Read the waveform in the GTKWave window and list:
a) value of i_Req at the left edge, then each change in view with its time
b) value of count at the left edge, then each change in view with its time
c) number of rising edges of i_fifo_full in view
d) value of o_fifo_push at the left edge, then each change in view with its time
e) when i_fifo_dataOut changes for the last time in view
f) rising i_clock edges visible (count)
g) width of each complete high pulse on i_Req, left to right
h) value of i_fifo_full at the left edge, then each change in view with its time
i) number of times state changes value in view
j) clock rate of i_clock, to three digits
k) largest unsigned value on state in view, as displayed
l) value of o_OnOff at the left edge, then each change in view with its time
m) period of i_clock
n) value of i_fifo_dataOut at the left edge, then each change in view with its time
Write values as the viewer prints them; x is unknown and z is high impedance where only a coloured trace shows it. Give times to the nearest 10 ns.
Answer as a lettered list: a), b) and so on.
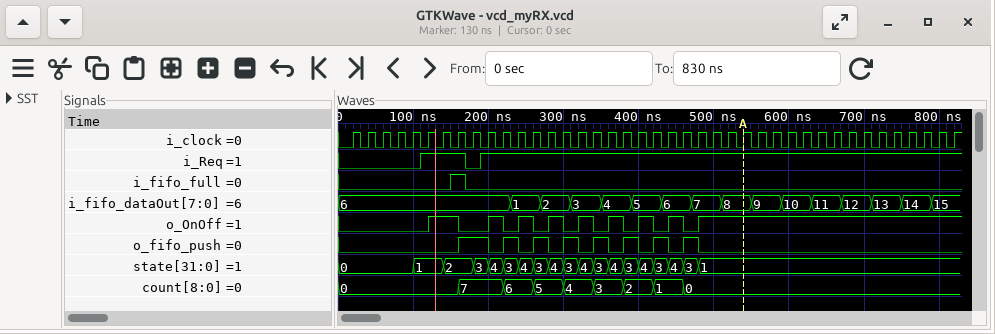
a) 0, 1 at 110 ns, 0 at 170 ns, 1 at 190 ns
b) 0, 7 at 160 ns, 6 at 220 ns, 5 at 260 ns, 4 at 300 ns, 3 at 340 ns, 2 at 380 ns, 1 at 420 ns, 0 at 460 ns
c) 1
d) 0, 1 at 160 ns, 0 at 200 ns, 1 at 220 ns, 0 at 240 ns, 1 at 260 ns, 0 at 280 ns, 1 at 300 ns, 0 at 320 ns, 1 at 340 ns, 0 at 360 ns, 1 at 380 ns, 0 at 400 ns, 1 at 420 ns, 0 at 440 ns, 1 at 460 ns, 0 at 480 ns
e) 790 ns
f) 41
g) 60 ns
h) 0, 1 at 150 ns, 0 at 170 ns
i) 18
j) 50.0 MHz
k) 4
l) 0, 1 at 120 ns, 0 at 160 ns, 1 at 200 ns, 0 at 220 ns, 1 at 240 ns, 0 at 260 ns, 1 at 280 ns, 0 at 300 ns, 1 at 320 ns, 0 at 340 ns, 1 at 360 ns, 0 at 380 ns, 1 at 400 ns, 0 at 420 ns, 1 at 440 ns, 0 at 460 ns, 1 at 480 ns
m) 20 ns
n) 6, 1 at 230 ns, 2 at 270 ns, 3 at 310 ns, 4 at 350 ns, 5 at 390 ns, 6 at 430 ns, 7 at 470 ns, 8 at 510 ns, 9 at 550 ns, 10 at 590 ns, 11 at 630 ns, 12 at 670 ns, 13 at 710 ns, 14 at 750 ns, 15 at 790 ns
